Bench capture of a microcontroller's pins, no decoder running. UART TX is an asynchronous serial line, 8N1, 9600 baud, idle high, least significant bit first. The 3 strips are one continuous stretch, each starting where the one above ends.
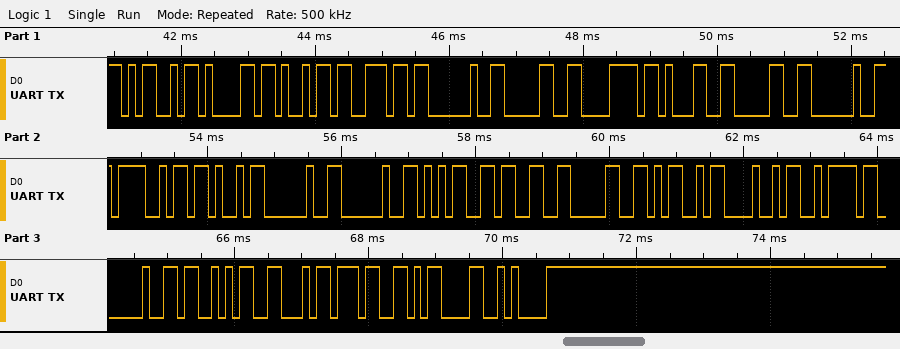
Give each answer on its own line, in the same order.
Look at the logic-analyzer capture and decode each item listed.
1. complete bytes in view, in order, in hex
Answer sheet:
4D 61 69 6E 20 30 78 31 30 20 4F 4B 20 20 35 33 30 4D 48 7A 20 53 46 37 0D 0A
